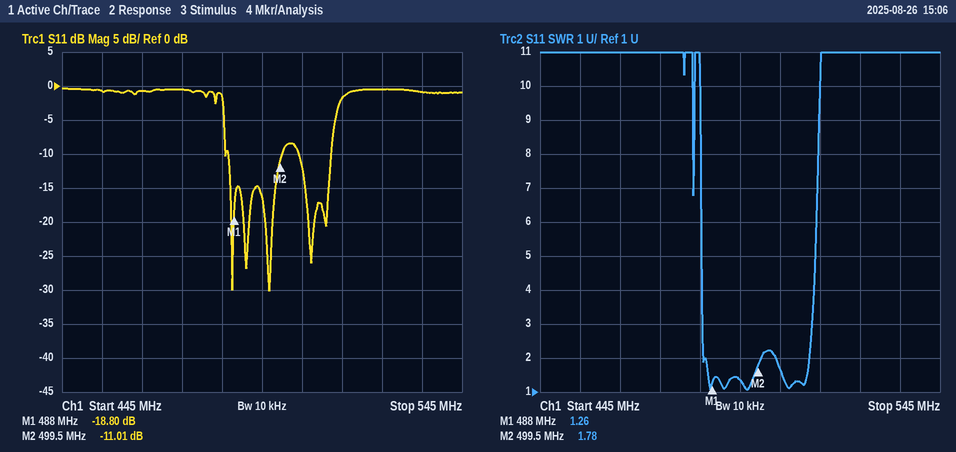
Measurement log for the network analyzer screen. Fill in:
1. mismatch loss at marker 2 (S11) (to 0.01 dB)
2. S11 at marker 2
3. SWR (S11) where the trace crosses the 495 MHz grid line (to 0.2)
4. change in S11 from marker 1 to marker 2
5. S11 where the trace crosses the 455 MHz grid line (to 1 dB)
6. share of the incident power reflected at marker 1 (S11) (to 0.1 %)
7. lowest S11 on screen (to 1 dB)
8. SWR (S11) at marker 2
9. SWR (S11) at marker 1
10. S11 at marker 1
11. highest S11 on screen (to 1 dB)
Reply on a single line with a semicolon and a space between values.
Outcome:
0.36 dB; -11.01 dB; 1.4; 7.79 dB; -1 dB; 1.3 %; -30 dB; 1.78; 1.26; -18.80 dB; 0 dB
